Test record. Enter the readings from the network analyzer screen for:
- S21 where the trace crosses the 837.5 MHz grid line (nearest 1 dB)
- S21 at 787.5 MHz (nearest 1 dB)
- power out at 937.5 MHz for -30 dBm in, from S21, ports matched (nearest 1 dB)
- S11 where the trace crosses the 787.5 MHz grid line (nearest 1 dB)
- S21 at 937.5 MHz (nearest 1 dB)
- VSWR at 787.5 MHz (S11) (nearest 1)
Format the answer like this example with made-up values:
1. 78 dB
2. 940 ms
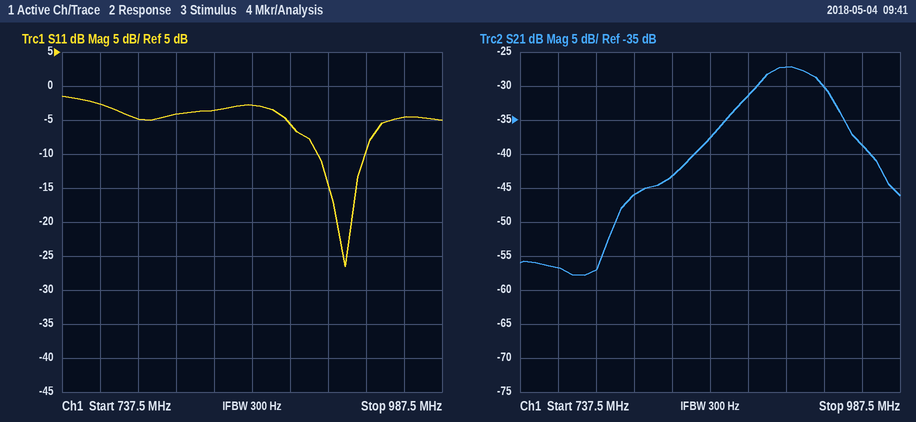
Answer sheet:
1. -43 dB
2. -57 dB
3. -60 dBm
4. -5 dB
5. -30 dB
6. 4
